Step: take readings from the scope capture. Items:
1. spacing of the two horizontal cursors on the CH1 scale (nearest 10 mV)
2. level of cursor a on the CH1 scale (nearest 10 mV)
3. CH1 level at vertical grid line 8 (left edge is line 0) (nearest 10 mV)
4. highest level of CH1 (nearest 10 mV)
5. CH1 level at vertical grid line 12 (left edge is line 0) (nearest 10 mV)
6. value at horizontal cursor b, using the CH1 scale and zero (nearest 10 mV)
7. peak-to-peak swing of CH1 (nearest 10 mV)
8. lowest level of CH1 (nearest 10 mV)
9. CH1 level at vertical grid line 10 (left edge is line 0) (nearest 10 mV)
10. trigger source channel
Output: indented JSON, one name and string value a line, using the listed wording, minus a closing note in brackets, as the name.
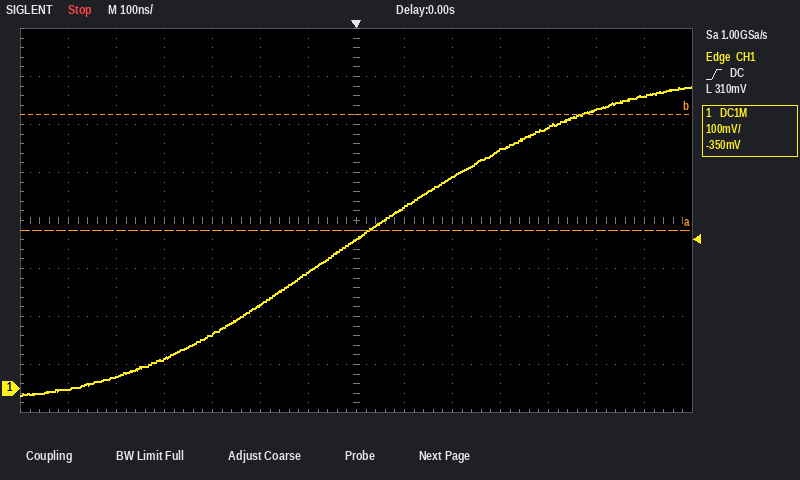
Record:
{
  "spacing of the two horizontal cursors on the CH1 scale": "240 mV",
  "level of cursor a on the CH1 scale": "330 mV",
  "CH1 level at vertical grid line 8 (left edge is line 0)": "380 mV",
  "highest level of CH1": "630 mV",
  "CH1 level at vertical grid line 12 (left edge is line 0)": "580 mV",
  "value at horizontal cursor b, using the CH1 scale and zero": "570 mV",
  "peak-to-peak swing of CH1": "640 mV",
  "lowest level of CH1": "-10 mV",
  "CH1 level at vertical grid line 10 (left edge is line 0)": "500 mV",
  "trigger source channel": "CH1"
}
